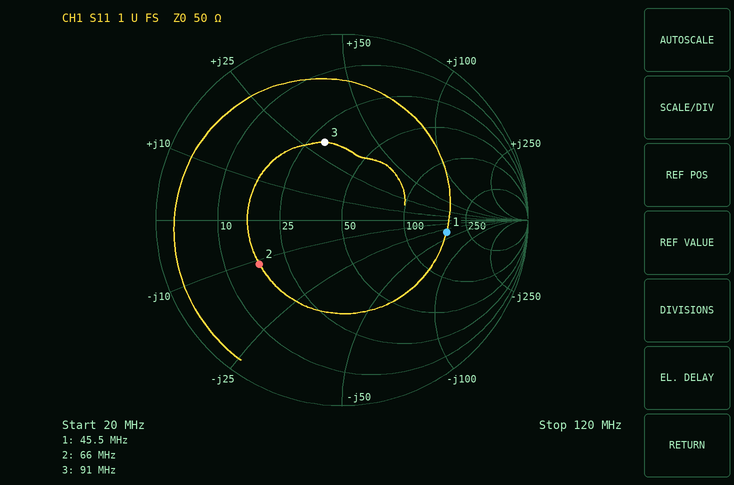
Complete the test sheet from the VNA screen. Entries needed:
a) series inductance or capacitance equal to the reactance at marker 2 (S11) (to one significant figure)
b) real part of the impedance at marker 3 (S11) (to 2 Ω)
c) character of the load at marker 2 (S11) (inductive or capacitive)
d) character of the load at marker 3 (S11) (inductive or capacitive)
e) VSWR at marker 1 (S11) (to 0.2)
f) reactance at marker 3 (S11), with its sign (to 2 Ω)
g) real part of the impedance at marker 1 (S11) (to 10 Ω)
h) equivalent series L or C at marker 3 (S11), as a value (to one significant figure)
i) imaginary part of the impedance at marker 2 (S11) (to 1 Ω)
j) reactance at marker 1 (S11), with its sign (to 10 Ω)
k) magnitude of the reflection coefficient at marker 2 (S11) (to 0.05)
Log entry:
200 pF
30 Ω
capacitive
inductive
3.6
+30 Ω
170 Ω
50 nH
-11 Ω
-30 Ω
0.50
